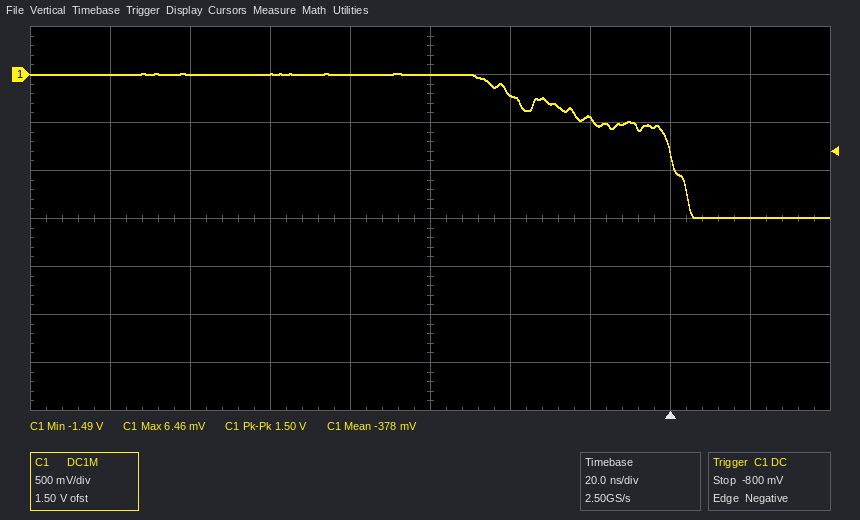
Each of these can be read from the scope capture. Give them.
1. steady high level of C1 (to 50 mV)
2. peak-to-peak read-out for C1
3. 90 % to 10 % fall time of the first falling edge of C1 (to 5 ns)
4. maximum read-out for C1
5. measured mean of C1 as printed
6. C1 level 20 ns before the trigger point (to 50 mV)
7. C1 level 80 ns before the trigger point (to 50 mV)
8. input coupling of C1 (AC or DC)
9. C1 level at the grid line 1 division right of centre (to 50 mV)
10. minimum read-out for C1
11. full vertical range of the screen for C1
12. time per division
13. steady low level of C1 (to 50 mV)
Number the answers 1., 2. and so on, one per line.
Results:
1. 0 mV
2. 1.50 V
3. 45 ns
4. 6.46 mV
5. -378 mV
6. -450 mV
7. 0 mV
8. DC
9. -200 mV
10. -1.49 V
11. 4 V
12. 20 ns
13. -1.50 V
